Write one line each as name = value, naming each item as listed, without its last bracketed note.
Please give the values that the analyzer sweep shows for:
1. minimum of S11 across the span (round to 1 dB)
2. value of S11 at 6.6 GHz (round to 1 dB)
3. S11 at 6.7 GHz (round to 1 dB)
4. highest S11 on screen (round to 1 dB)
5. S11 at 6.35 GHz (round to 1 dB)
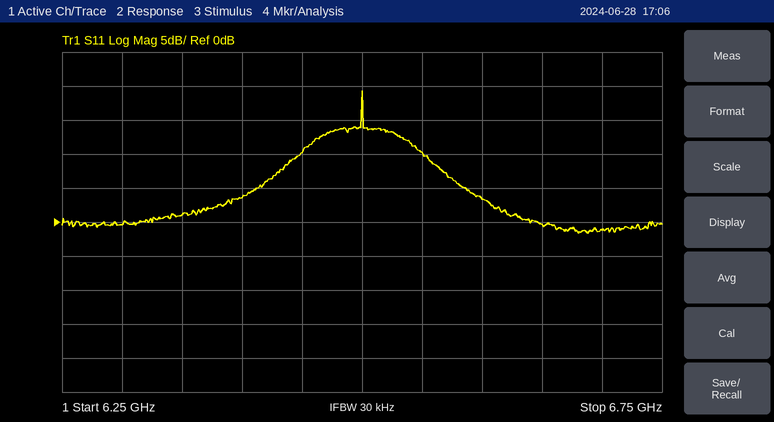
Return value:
minimum of S11 across the span = -2 dB
value of S11 at 6.6 GHz = 3 dB
S11 at 6.7 GHz = -1 dB
highest S11 on screen = 19 dB
S11 at 6.35 GHz = 1 dB
